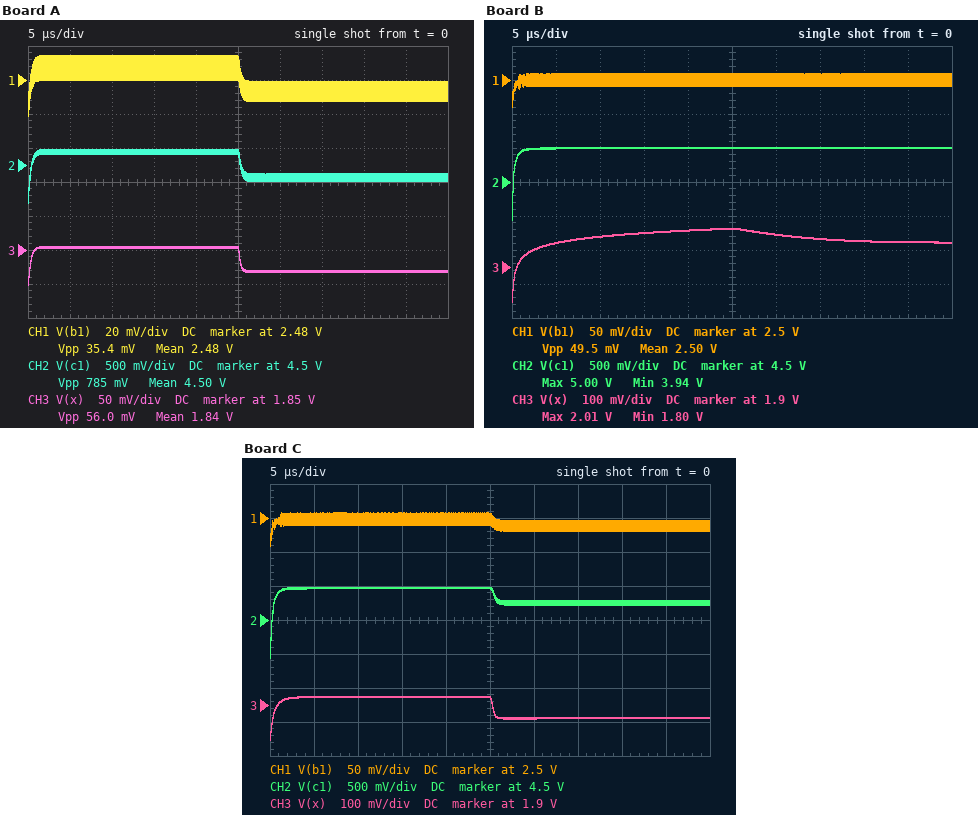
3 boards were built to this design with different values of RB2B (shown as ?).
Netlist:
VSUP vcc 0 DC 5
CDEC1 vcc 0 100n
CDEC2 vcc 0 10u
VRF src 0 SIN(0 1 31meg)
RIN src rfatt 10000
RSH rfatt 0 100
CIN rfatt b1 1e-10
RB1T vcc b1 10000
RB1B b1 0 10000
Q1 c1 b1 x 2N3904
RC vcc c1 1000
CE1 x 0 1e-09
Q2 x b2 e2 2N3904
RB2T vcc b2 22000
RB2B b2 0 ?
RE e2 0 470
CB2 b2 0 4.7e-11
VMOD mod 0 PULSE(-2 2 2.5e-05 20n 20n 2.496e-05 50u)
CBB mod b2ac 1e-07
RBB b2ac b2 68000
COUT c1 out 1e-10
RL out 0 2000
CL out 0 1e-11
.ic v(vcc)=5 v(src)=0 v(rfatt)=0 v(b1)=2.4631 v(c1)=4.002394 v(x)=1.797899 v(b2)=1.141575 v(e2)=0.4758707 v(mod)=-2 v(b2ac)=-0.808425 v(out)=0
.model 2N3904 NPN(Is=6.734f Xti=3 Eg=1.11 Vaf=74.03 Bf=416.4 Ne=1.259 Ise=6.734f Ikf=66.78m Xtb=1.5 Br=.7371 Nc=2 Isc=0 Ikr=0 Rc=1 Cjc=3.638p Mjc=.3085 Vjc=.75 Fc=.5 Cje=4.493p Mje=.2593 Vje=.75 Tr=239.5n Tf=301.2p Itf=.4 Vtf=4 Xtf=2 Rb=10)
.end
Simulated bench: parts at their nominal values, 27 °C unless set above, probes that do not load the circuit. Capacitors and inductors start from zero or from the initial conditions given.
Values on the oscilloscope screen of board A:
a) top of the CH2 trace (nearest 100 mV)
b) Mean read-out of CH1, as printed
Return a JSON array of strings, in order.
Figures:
["4.7 V", "2.48 V"]
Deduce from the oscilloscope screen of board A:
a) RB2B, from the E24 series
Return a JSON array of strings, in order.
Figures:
["4.7 kΩ"]
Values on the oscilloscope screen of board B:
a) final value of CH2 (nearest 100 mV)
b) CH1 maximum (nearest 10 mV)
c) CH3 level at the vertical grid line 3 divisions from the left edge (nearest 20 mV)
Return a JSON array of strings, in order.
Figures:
["5.0 V", "2.51 V", "2.00 V"]
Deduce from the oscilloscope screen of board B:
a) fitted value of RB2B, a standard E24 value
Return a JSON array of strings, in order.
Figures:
["2.2 kΩ"]
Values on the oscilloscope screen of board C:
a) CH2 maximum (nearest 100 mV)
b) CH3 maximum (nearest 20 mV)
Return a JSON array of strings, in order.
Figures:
["5.0 V", "1.92 V"]
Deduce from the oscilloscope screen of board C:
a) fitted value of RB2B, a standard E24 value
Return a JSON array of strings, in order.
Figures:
["3.3 kΩ"]
